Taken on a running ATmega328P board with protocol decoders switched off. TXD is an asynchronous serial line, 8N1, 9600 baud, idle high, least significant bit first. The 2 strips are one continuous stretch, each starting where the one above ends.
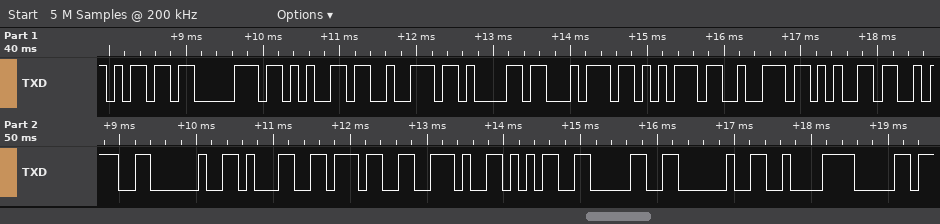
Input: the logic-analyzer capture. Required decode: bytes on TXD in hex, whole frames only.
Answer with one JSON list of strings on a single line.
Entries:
["0x6D 0x70 0x65 0x72 0x61 0x74 0x75 0x72 0x65 0x3A 0x20 0x31 0x37 0x2E 0x35 0x30 0x20 0xC2 0xB0"]
